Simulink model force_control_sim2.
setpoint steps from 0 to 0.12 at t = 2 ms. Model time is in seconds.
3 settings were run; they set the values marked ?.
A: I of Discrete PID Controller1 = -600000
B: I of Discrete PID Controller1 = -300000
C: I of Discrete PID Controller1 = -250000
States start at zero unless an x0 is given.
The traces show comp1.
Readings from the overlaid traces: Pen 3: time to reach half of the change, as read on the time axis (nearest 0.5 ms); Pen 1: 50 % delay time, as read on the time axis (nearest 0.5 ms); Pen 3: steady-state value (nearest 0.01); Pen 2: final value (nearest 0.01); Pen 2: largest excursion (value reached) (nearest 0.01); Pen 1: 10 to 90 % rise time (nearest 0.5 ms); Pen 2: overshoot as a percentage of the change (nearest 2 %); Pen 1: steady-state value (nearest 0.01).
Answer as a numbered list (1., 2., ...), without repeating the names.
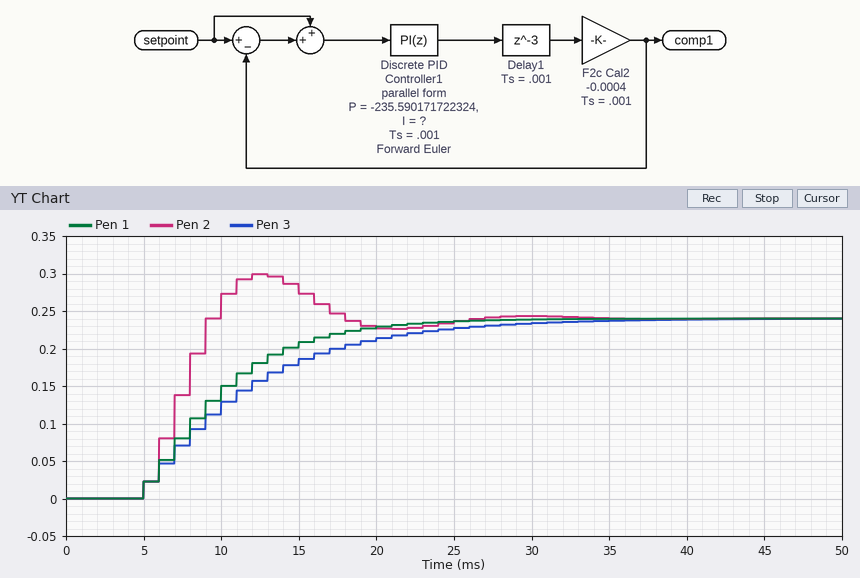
1. 10.0 ms
2. 9.0 ms
3. 0.24
4. 0.24
5. 0.30
6. 11.0 ms
7. 24 %
8. 0.24
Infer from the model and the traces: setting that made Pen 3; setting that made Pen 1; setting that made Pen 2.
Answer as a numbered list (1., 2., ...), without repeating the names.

1. C
2. B
3. A
